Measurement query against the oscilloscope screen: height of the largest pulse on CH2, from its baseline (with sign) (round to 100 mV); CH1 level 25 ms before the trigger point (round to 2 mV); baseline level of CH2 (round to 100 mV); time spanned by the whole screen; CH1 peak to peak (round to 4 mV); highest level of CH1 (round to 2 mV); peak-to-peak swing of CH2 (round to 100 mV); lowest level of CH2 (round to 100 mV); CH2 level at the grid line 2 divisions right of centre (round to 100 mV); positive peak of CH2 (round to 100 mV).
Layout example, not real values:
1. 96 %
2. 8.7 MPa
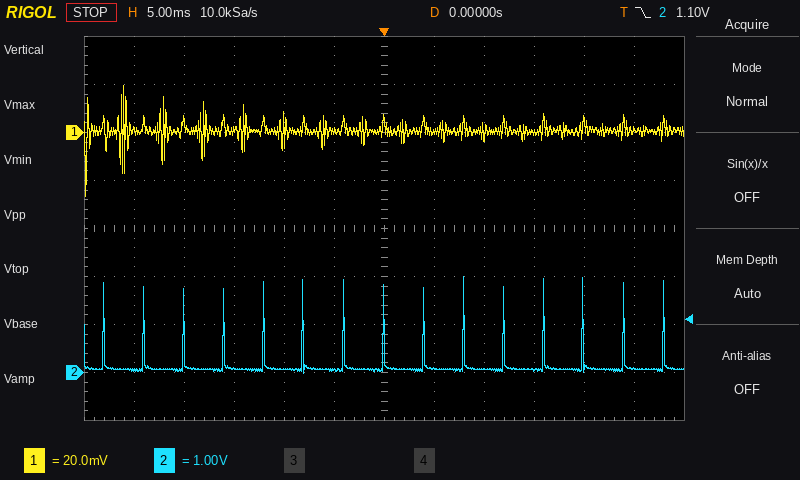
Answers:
1. +1.9 V
2. 0 mV
3. 100 mV
4. 60 ms
5. 48 mV
6. 20 mV
7. 2.0 V
8. 0.0 V
9. 100 mV
10. 2.0 V
